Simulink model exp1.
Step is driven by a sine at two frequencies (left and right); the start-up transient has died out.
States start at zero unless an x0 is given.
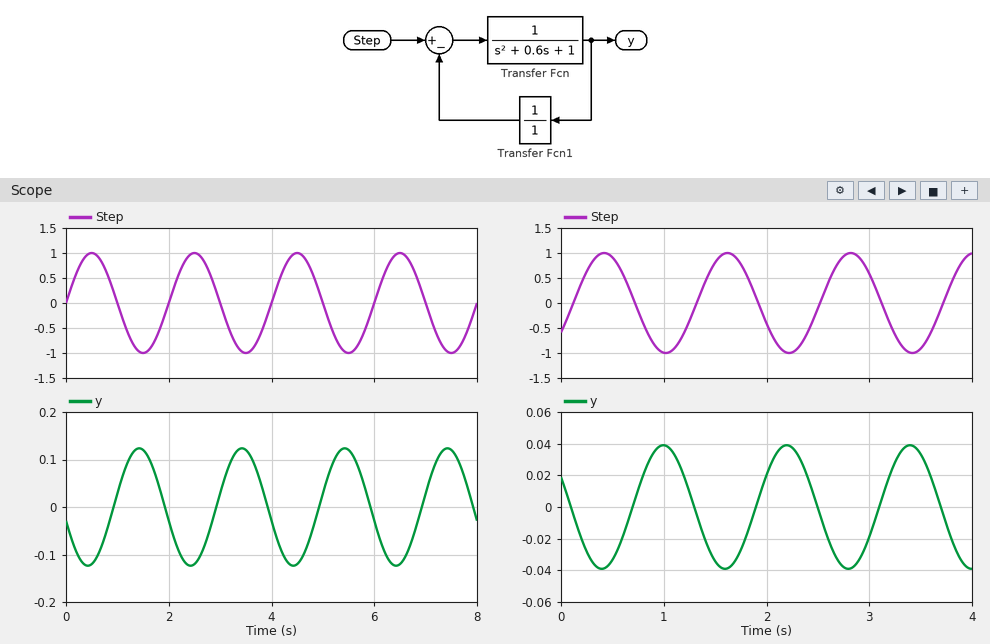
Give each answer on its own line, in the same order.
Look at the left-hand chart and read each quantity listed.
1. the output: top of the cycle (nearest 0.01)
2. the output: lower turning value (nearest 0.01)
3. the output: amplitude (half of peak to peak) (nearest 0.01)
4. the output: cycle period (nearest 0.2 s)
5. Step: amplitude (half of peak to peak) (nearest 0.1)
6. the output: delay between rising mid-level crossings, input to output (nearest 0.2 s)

0.12
-0.12
0.12
2.0 s
1.0
1.0 s
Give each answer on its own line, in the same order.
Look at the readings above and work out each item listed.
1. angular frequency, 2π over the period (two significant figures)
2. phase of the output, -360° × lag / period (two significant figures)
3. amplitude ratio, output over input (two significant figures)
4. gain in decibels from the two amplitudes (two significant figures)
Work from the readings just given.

3.1 rad/s
-180°
0.12
-18 dB
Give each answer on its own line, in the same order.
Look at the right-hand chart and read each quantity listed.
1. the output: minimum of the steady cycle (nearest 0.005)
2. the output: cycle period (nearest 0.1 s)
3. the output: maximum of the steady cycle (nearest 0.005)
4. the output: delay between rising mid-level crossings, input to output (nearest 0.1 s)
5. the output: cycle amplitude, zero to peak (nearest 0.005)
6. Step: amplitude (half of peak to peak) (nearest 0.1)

-0.040
1.2 s
0.040
0.6 s
0.040
1.0
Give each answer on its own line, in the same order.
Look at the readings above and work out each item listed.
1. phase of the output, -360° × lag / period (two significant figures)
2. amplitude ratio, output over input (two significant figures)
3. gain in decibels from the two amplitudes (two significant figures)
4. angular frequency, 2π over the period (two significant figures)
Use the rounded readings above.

-180°
0.040
-28 dB
5.2 rad/s
